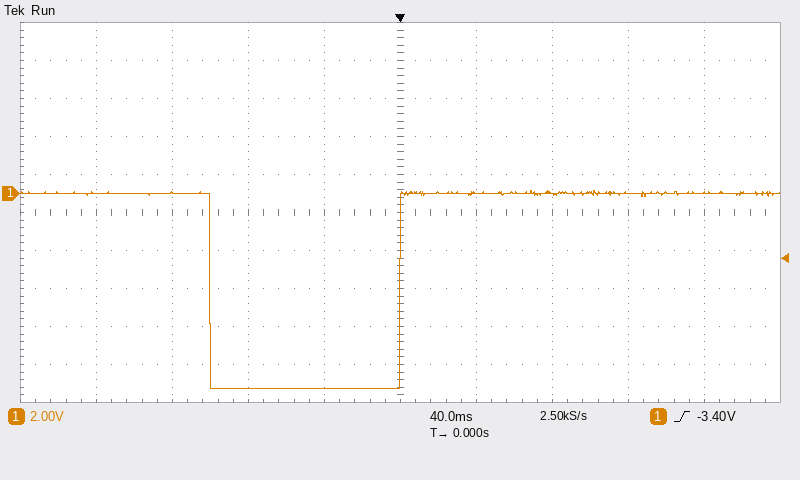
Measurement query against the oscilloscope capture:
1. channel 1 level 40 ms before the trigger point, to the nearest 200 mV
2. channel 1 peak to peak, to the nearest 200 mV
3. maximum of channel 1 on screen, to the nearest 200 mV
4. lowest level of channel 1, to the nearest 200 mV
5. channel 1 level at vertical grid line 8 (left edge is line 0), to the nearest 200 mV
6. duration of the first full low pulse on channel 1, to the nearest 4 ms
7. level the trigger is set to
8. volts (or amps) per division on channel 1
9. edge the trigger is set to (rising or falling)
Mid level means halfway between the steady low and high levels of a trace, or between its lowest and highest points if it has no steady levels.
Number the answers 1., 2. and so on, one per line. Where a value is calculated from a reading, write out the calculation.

1. -10.2 V
2. 200 mV − (-10.2 V) = 10.4 V
3. 200 mV
4. -10.2 V
5. 0.0 V
6. 100 ms
7. -3.40 V
8. 2 V
9. rising
